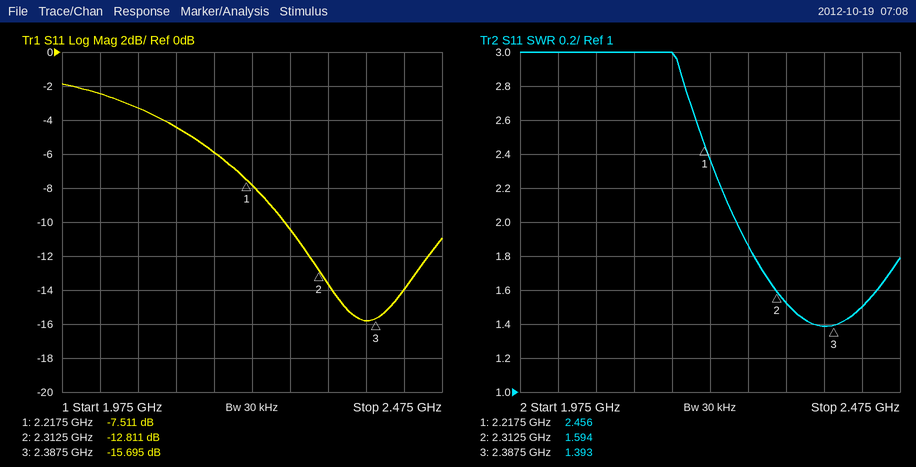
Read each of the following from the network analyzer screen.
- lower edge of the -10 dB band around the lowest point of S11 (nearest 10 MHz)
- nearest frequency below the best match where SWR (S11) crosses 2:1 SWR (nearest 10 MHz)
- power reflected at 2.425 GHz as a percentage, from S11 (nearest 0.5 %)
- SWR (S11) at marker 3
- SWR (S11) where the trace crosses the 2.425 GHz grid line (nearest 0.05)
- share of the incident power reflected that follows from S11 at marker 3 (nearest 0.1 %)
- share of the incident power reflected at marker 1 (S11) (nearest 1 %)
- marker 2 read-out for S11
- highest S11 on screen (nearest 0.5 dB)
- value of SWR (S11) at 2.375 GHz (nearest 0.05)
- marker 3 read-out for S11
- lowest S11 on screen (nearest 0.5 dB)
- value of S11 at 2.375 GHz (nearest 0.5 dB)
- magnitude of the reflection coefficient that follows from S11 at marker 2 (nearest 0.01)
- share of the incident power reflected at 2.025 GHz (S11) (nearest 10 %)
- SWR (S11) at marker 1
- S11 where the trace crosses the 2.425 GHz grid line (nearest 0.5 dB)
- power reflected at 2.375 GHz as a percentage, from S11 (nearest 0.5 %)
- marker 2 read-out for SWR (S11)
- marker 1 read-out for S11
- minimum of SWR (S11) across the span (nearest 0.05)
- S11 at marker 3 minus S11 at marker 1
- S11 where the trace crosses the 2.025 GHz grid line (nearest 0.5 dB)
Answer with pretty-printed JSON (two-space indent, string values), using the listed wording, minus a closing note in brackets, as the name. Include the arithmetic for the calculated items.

{
  "lower edge of the -10 dB band around the lowest point of S11": "2.27 GHz",
  "nearest frequency below the best match where SWR (S11) crosses 2:1 SWR": "2.26 GHz",
  "power reflected at 2.425 GHz as a percentage, from S11": "10^(-14/10) ≈ 4.0 %",
  "SWR (S11) at marker 3": "1.393",
  "SWR (S11) where the trace crosses the 2.425 GHz grid line": "1.50",
  "share of the incident power reflected that follows from S11 at marker 3": "10^(-15.695/10) ≈ 2.7 %",
  "share of the incident power reflected at marker 1 (S11)": "10^(-7.511/10) ≈ 18 %",
  "marker 2 read-out for S11": "-12.811 dB",
  "highest S11 on screen": "-2.0 dB",
  "value of SWR (S11) at 2.375 GHz": "1.40",
  "marker 3 read-out for S11": "-15.695 dB",
  "lowest S11 on screen": "-16.0 dB",
  "value of S11 at 2.375 GHz": "-16.0 dB",
  "magnitude of the reflection coefficient that follows from S11 at marker 2": "10^(-12.811/20) ≈ 0.23",
  "share of the incident power reflected at 2.025 GHz (S11)": "10^(-2.5/10) ≈ 56.2 %, so 60 % to the nearest 10 %",
  "SWR (S11) at marker 1": "2.456",
  "S11 where the trace crosses the 2.425 GHz grid line": "-14.0 dB",
  "power reflected at 2.375 GHz as a percentage, from S11": "10^(-16/10) ≈ 2.5 %",
  "marker 2 read-out for SWR": "1.594",
  "marker 1 read-out for S11": "-7.511 dB",
  "minimum of SWR (S11) across the span": "1.40",
  "S11 at marker 3 minus S11 at marker 1": "-15.695 − (-7.511) = -8.184 dB",
  "S11 where the trace crosses the 2.025 GHz grid line": "-2.5 dB"
}
